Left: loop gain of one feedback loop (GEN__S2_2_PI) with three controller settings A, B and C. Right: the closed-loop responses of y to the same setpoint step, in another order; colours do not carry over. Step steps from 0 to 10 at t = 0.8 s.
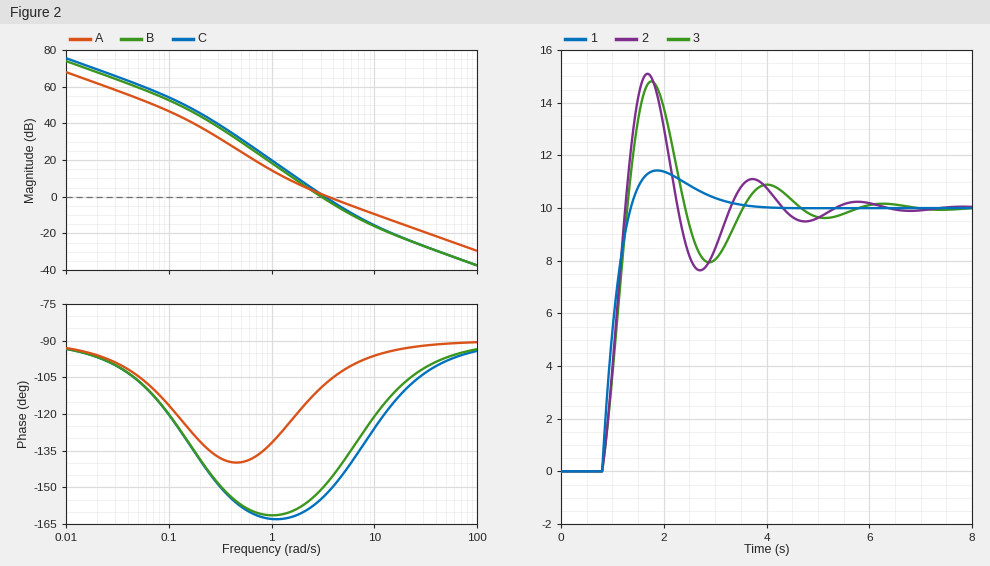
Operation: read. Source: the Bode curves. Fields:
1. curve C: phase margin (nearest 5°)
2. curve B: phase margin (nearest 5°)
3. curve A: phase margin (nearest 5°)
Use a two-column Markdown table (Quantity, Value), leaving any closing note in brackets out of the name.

| Quantity | Value |
|---|---|
| curve C: phase margin | 25° |
| curve B: phase margin | 30° |
| curve A: phase margin | 75° |
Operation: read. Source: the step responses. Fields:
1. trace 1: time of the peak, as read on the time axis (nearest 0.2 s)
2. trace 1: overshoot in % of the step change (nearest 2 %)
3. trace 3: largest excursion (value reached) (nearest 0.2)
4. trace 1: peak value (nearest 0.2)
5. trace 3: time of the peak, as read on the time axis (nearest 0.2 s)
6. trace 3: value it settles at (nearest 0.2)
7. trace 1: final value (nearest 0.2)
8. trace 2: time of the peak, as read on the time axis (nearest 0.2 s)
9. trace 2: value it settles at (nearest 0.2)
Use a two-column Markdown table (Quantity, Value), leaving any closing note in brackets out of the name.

| Quantity | Value |
|---|---|
| trace 1: time of the peak, as read on the time axis | 1.8 s |
| trace 1: overshoot in % of the step change | 14 % |
| trace 3: largest excursion (value reached) | 14.8 |
| trace 1: peak value | 11.4 |
| trace 3: time of the peak, as read on the time axis | 1.8 s |
| trace 3: value it settles at | 10.0 |
| trace 1: final value | 10.0 |
| trace 2: time of the peak, as read on the time axis | 1.6 s |
| trace 2: value it settles at | 10.0 |
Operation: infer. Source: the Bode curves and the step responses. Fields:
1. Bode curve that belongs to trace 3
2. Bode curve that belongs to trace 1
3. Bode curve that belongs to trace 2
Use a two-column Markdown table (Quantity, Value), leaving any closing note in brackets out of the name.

| Quantity | Value |
|---|---|
| Bode curve that belongs to trace 3 | B |
| Bode curve that belongs to trace 1 | A |
| Bode curve that belongs to trace 2 | C |
